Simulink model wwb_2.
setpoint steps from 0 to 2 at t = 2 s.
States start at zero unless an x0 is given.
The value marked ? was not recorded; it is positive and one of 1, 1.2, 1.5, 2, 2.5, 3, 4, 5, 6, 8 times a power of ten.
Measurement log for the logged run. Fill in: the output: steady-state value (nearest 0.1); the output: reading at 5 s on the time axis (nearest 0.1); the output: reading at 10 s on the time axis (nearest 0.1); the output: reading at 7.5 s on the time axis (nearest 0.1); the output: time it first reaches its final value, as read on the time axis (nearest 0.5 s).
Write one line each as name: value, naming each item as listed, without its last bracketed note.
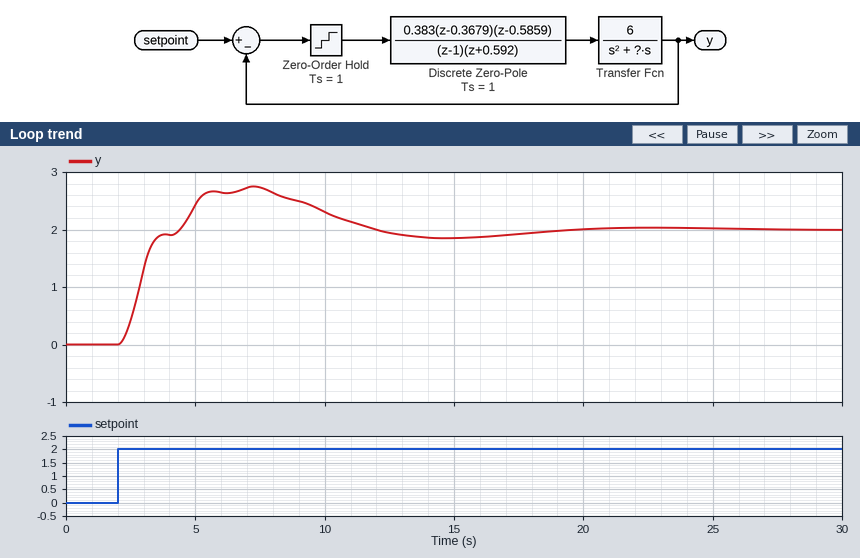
the output: steady-state value: 2.0
the output: reading at 5 s on the time axis: 2.4
the output: reading at 10 s on the time axis: 2.3
the output: reading at 7.5 s on the time axis: 2.7
the output: time it first reaches its final value, as read on the time axis: 4.5 s
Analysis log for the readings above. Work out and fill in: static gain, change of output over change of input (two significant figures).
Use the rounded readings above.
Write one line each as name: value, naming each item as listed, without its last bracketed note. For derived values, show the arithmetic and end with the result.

static gain, change of output over change of input: (2 - 0) / (2 - 0) = 1.0
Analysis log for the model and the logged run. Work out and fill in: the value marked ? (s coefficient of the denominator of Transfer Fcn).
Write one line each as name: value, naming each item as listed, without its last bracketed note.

the value marked ?: 2
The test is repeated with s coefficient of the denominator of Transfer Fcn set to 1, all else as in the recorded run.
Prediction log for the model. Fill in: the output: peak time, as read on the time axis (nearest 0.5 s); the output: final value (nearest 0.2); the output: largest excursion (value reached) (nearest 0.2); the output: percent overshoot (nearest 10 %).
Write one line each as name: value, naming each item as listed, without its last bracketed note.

the output: peak time, as read on the time axis: 5.0 s
the output: final value: 2.0
the output: largest excursion (value reached): 3.0
the output: percent overshoot: 50 %
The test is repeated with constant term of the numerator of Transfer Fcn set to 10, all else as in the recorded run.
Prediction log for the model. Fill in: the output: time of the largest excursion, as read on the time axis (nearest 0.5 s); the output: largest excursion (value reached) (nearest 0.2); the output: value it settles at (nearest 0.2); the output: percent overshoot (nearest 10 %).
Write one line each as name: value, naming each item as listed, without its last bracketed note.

the output: time of the largest excursion, as read on the time axis: 5.5 s
the output: largest excursion (value reached): 2.8
the output: value it settles at: 2.0
the output: percent overshoot: 40 %
